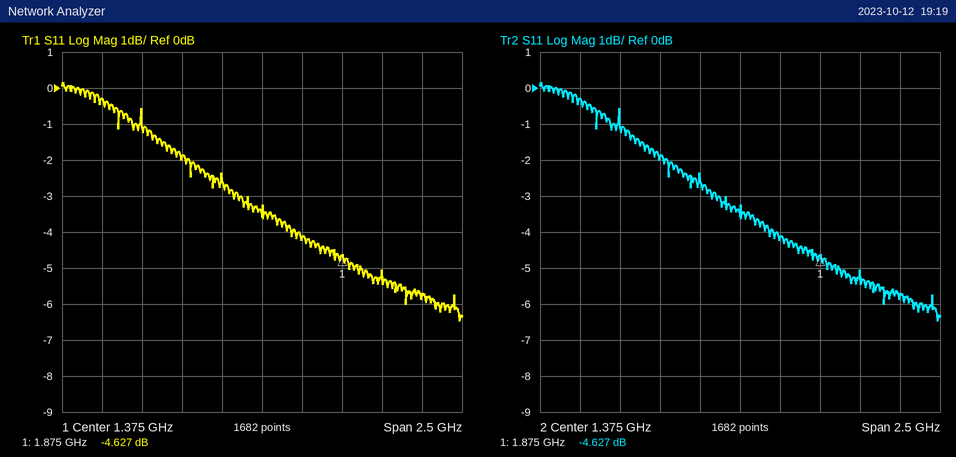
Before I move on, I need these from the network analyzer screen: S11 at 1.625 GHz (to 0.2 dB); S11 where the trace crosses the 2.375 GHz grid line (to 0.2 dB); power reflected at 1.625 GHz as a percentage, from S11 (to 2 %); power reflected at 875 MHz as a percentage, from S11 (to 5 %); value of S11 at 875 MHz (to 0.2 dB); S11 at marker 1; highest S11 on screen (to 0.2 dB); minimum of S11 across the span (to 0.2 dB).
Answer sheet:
-4.2 dB
-5.8 dB
38 %
65 %
-2.0 dB
-4.627 dB
0.2 dB
-6.4 dB
